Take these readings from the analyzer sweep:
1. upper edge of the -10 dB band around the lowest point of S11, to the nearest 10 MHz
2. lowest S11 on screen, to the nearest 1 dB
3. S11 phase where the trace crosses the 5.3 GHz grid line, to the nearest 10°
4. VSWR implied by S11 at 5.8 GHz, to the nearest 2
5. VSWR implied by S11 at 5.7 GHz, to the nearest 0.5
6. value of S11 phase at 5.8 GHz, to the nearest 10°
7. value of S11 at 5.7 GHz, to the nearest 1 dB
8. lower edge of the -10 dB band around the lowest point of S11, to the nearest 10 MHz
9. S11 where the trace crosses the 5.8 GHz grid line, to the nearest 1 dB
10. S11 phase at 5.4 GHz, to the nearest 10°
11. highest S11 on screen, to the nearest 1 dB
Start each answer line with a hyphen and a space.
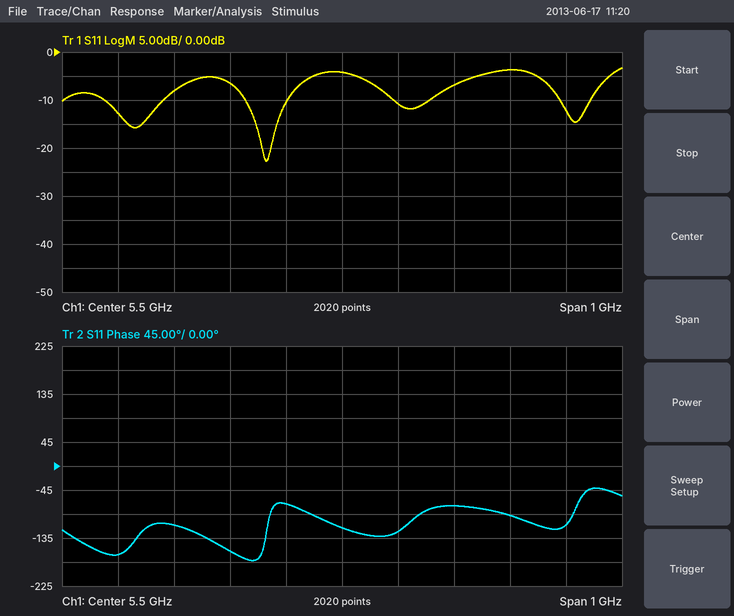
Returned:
- 5.40 GHz
- -23 dB
- -160°
- 4
- 2.5
- -90°
- -7 dB
- 5.33 GHz
- -4 dB
- -70°
- -3 dB
